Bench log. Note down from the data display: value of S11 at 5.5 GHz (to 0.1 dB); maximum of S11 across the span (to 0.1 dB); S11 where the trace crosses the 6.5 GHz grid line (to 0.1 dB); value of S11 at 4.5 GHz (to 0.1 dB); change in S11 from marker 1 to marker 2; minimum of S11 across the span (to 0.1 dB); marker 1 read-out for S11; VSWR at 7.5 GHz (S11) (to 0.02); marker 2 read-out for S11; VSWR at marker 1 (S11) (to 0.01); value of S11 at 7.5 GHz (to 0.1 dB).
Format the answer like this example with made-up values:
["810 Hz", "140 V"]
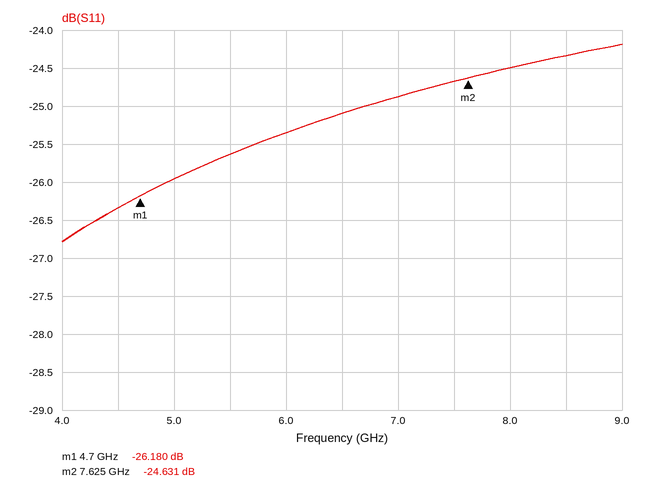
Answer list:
["-25.6 dB", "-24.2 dB", "-25.1 dB", "-26.3 dB", "1.549 dB", "-26.8 dB", "-26.180 dB", "1.12", "-24.631 dB", "1.10", "-24.7 dB"]
